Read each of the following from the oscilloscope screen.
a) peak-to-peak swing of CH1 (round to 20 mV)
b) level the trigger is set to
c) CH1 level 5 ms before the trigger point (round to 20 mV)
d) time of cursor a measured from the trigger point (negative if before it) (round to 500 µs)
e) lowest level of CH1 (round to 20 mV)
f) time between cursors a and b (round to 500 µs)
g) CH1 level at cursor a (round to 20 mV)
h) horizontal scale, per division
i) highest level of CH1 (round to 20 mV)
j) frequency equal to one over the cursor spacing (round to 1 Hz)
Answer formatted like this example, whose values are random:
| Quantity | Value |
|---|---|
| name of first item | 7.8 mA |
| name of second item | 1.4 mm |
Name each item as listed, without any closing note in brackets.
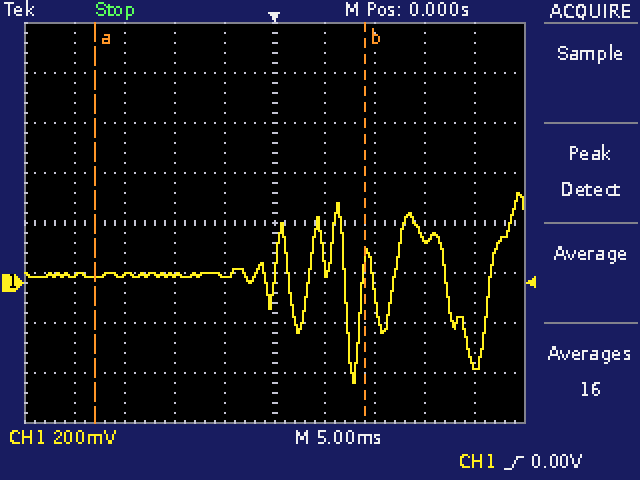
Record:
| Quantity | Value |
|---|---|
| peak-to-peak swing of CH1 | 760 mV |
| level the trigger is set to | 0.00 V |
| CH1 level 5 ms before the trigger point | 20 mV |
| time of cursor a measured from the trigger point (negative if before it) | -18.0 ms |
| lowest level of CH1 | -400 mV |
| time between cursors a and b | 27.0 ms |
| CH1 level at cursor a | 20 mV |
| horizontal scale, per division | 5 ms |
| highest level of CH1 | 360 mV |
| frequency equal to one over the cursor spacing | 37 Hz |
